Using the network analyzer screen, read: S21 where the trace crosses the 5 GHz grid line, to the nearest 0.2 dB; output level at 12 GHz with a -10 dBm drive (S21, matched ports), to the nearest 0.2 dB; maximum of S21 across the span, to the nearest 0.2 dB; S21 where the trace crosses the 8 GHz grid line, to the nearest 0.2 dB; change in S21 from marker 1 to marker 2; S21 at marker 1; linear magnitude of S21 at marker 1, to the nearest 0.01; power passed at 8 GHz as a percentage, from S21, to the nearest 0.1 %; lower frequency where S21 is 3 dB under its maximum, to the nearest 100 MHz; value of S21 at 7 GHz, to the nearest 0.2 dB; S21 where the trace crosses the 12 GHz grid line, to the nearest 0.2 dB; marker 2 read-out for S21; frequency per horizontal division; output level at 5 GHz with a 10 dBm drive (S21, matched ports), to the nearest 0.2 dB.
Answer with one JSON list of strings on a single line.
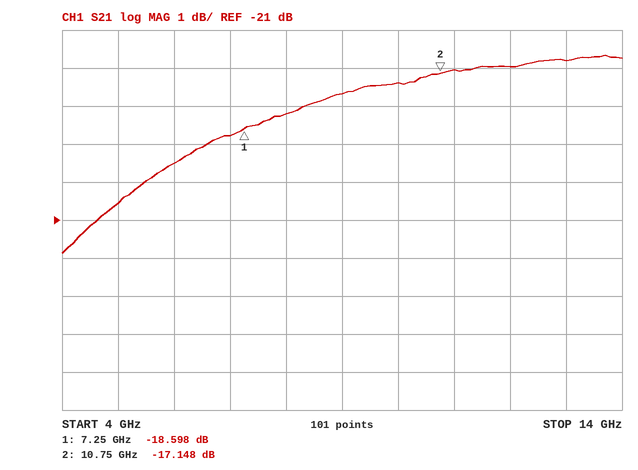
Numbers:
["-20.6 dB", "-27.0 dBm", "-16.6 dB", "-18.2 dB", "1.450 dB", "-18.598 dB", "0.12", "1.5 %", "5.8 GHz", "-18.8 dB", "-17.0 dB", "-17.148 dB", "1 GHz", "-10.6 dBm"]
